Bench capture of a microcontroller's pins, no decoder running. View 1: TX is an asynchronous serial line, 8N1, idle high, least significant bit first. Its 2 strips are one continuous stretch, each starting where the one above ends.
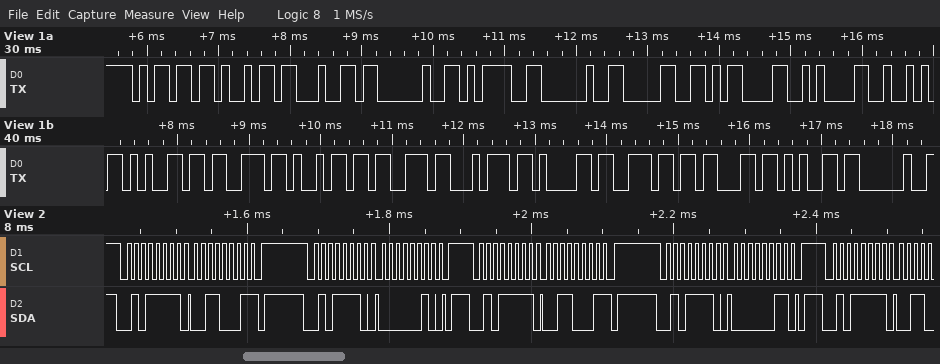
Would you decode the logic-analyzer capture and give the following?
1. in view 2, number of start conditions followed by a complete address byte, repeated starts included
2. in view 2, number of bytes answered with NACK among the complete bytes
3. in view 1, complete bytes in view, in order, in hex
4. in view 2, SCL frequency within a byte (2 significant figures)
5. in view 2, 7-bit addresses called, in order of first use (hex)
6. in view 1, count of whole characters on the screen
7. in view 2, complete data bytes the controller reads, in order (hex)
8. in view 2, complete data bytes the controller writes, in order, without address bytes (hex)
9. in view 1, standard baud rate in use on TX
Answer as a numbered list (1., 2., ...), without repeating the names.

1. 5
2. 2
3. 6D 69 64 20 3D 20 30 0D 0A 52 65 73 69 73 74 61 6E 63 65 20
4. 100 kHz
5. 0x2F
6. 20
7. 31 31
8. 02 03
9. 9600 baud
